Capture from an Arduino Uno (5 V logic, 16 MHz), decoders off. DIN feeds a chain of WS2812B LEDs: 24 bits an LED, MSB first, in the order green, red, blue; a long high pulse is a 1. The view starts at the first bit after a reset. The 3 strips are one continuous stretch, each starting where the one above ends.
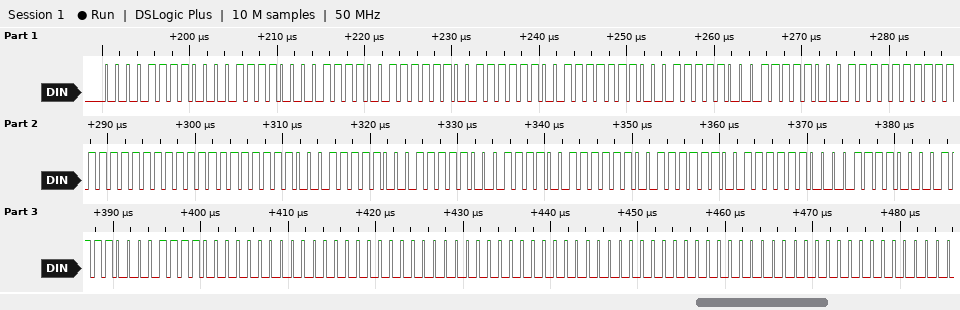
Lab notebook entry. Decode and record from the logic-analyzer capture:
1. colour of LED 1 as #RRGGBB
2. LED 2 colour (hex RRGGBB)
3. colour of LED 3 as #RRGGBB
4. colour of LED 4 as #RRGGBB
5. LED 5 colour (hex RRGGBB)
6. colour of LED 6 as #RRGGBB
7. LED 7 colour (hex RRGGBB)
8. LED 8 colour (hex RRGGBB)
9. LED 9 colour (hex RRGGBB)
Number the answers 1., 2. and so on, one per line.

1. #0F0F0F
2. #3F3F3F
3. #8F8F8F
4. #FFFFFF
5. #8F8F8F
6. #3F3F3F
7. #0F0F0F
8. #000000
9. #000000
